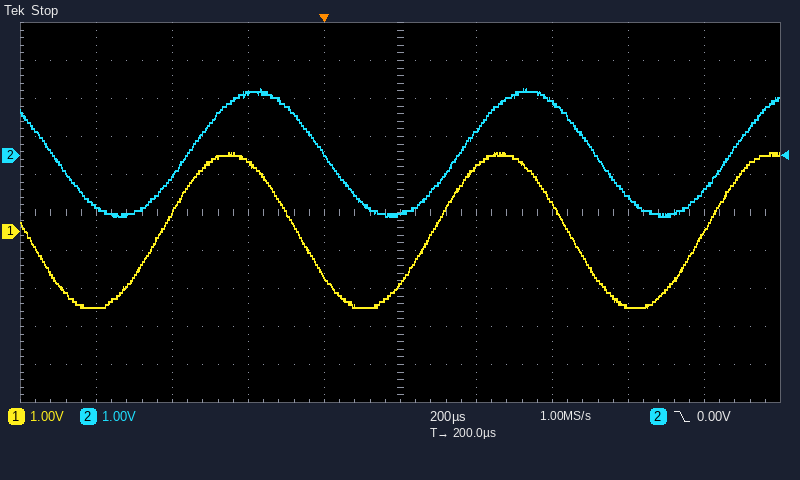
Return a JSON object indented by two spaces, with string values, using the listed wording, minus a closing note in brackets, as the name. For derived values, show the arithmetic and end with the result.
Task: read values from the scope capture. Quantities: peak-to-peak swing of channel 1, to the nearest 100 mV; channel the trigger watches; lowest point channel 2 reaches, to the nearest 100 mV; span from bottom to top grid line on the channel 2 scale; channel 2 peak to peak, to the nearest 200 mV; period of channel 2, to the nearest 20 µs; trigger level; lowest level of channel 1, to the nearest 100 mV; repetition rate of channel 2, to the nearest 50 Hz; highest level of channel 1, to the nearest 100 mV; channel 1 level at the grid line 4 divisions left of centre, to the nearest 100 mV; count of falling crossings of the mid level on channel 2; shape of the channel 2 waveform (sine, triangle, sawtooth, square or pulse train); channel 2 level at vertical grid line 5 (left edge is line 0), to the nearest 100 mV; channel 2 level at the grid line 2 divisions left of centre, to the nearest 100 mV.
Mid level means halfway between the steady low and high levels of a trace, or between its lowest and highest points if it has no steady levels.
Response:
{
  "peak-to-peak swing of channel 1, to the nearest 100 mV": "2.1 V − (-2.0 V) = 4.1 V",
  "channel the trigger watches": "channel 2",
  "lowest point channel 2 reaches, to the nearest 100 mV": "-1.6 V",
  "span from bottom to top grid line on the channel 2 scale": "10 V",
  "channel 2 peak to peak, to the nearest 200 mV": "3.4 V",
  "period of channel 2, to the nearest 20 µs": "720 µs",
  "trigger level": "0.00 V",
  "lowest level of channel 1, to the nearest 100 mV": "-2.0 V",
  "repetition rate of channel 2, to the nearest 50 Hz": "1 / 720 µs ≈ 1.39 kHz, so 1.40 kHz to the nearest 50 Hz",
  "highest level of channel 1, to the nearest 100 mV": "2.1 V",
  "channel 1 level at the grid line 4 divisions left of centre, to the nearest 100 mV": "-2.0 V",
  "count of falling crossings of the mid level on channel 2": "3",
  "shape of the channel 2 waveform": "sine",
  "channel 2 level at vertical grid line 5 (left edge is line 0), to the nearest 100 mV": "-1.5 V",
  "channel 2 level at the grid line 2 divisions left of centre, to the nearest 100 mV": "1.6 V"
}
